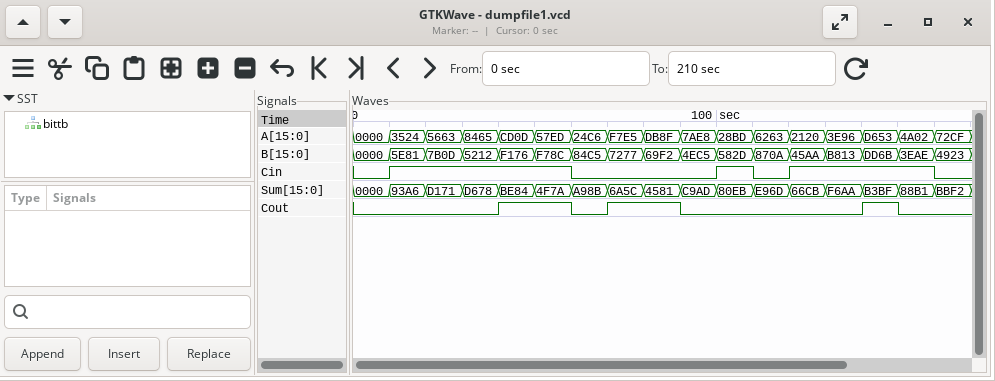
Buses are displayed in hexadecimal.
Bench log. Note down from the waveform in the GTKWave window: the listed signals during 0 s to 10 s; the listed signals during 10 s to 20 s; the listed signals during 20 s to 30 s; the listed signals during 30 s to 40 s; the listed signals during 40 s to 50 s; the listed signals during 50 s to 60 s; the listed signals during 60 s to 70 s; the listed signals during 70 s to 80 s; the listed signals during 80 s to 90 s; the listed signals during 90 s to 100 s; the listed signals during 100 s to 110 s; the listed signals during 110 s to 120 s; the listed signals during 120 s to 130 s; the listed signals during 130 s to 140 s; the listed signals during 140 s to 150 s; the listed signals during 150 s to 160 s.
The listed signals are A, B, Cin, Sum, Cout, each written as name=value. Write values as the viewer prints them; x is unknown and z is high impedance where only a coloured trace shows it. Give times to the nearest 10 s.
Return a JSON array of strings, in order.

["A=0000, B=0000, Cin=0, Sum=0000, Cout=0", "A=3524, B=5E81, Cin=1, Sum=93A6, Cout=0", "A=5663, B=7B0D, Cin=1, Sum=D171, Cout=0", "A=8465, B=5212, Cin=1, Sum=D678, Cout=0", "A=CD0D, B=F176, Cin=1, Sum=BE84, Cout=1", "A=57ED, B=F78C, Cin=1, Sum=4F7A, Cout=1", "A=24C6, B=84C5, Cin=0, Sum=A98B, Cout=0", "A=F7E5, B=7277, Cin=0, Sum=6A5C, Cout=1", "A=DB8F, B=69F2, Cin=0, Sum=4581, Cout=1", "A=7AE8, B=4EC5, Cin=0, Sum=C9AD, Cout=0", "A=28BD, B=582D, Cin=1, Sum=80EB, Cout=0", "A=6263, B=870A, Cin=0, Sum=E96D, Cout=0", "A=2120, B=45AA, Cin=1, Sum=66CB, Cout=0", "A=3E96, B=B813, Cin=1, Sum=F6AA, Cout=0", "A=D653, B=DD6B, Cin=1, Sum=B3BF, Cout=1", "A=4A02, B=3EAE, Cin=1, Sum=88B1, Cout=0"]
